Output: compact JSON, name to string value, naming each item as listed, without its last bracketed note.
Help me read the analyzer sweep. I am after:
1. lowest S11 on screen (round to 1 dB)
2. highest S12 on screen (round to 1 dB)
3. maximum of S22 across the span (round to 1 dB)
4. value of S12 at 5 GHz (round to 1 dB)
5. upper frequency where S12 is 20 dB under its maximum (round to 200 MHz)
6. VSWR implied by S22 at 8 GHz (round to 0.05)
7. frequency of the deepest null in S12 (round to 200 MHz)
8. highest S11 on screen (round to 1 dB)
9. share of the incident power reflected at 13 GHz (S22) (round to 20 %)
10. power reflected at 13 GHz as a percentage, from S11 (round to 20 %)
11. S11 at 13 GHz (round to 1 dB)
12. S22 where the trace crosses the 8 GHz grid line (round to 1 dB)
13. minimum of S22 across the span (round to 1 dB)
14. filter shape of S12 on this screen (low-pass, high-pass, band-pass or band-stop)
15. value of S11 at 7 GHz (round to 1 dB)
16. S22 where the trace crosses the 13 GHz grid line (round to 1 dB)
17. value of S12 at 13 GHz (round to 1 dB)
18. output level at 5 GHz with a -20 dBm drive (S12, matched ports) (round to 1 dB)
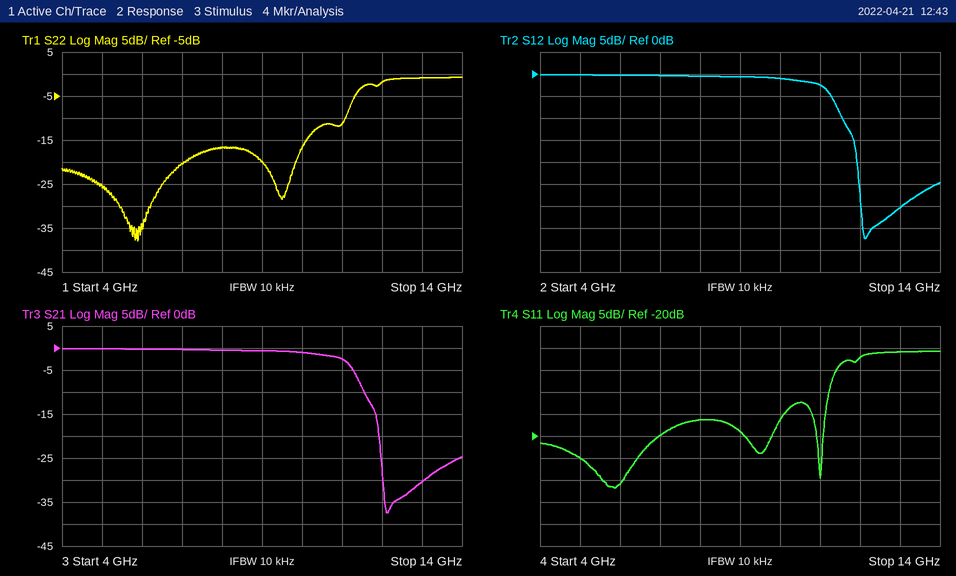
{"lowest S11 on screen": "-32 dB", "highest S12 on screen": "0 dB", "maximum of S22 across the span": "-1 dB", "value of S12 at 5 GHz": "0 dB", "upper frequency where S12 is 20 dB under its maximum": "12.0 GHz", "VSWR implied by S22 at 8 GHz": "1.35", "frequency of the deepest null in S12": "12.2 GHz", "highest S11 on screen": "-1 dB", "share of the incident power reflected at 13 GHz (S22)": "80 %", "power reflected at 13 GHz as a percentage, from S11": "80 %", "S11 at 13 GHz": "-1 dB", "S22 where the trace crosses the 8 GHz grid line": "-17 dB", "minimum of S22 across the span": "-38 dB", "filter shape of S12 on this screen": "low-pass", "value of S11 at 7 GHz": "-20 dB", "S22 where the trace crosses the 13 GHz grid line": "-1 dB", "value of S12 at 13 GHz": "-30 dB", "output level at 5 GHz with a -20 dBm drive (S12, matched ports)": "-20 dBm"}
